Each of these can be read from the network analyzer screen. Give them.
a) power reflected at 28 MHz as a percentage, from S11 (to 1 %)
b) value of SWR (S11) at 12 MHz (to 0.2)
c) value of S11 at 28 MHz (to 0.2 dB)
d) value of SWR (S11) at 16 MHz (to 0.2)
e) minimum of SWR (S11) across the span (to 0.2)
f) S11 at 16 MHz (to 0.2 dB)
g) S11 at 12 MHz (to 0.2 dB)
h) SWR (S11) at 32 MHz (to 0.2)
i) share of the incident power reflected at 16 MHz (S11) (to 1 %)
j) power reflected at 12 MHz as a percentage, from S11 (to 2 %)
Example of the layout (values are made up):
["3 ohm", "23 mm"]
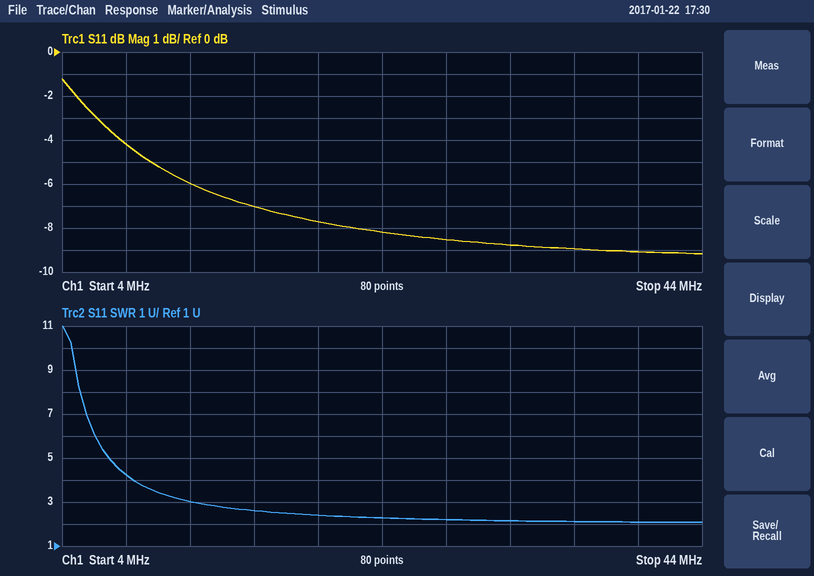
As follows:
["14 %", "3.0", "-8.6 dB", "2.6", "2.0", "-7.0 dB", "-6.0 dB", "2.2", "20 %", "26 %"]
